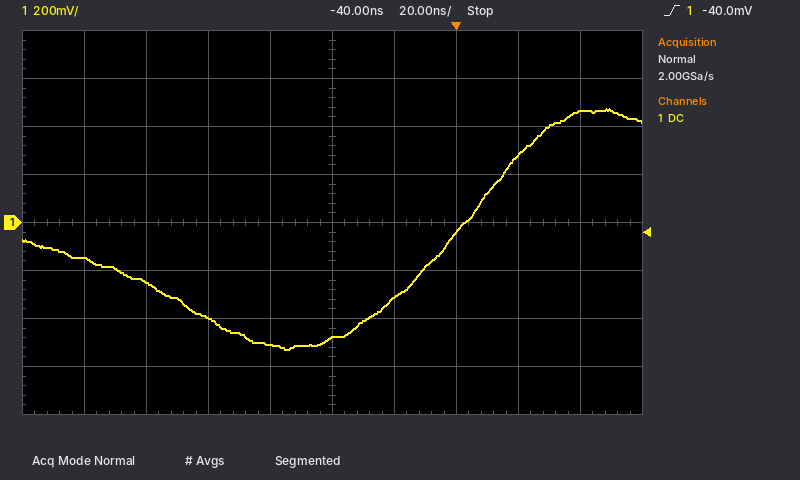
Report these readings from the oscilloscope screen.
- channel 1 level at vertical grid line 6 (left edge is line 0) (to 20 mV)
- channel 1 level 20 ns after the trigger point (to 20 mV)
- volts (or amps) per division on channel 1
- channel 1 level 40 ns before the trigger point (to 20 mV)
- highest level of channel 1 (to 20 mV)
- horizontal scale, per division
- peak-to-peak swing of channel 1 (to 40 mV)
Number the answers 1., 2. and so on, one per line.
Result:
1. -320 mV
2. 280 mV
3. 200 mV
4. -480 mV
5. 480 mV
6. 20 ns
7. 1.00 V
